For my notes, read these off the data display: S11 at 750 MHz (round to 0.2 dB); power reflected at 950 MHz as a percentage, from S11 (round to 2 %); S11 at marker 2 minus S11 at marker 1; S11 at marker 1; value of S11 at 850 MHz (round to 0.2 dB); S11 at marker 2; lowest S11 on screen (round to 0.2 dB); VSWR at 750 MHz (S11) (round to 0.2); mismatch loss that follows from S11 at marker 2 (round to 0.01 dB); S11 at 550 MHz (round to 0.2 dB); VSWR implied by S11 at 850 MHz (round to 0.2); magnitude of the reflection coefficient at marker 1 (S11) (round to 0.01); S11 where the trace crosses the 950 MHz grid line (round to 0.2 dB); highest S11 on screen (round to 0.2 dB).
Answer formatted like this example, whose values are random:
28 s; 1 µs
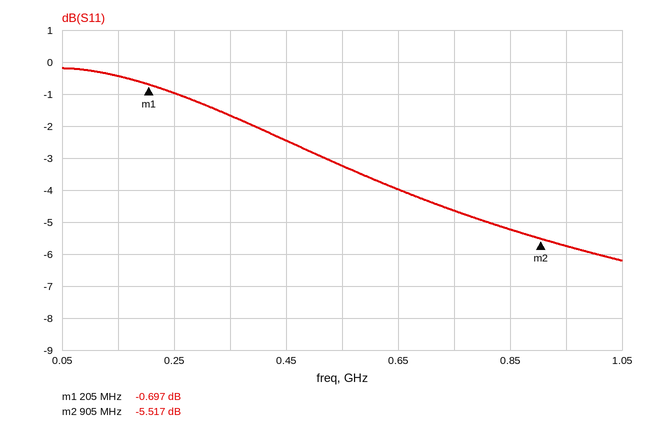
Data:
-4.6 dB; 26 %; -4.820 dB; -0.697 dB; -5.2 dB; -5.517 dB; -6.2 dB; 3.8; 1.43 dB; -3.2 dB; 3.4; 0.92; -5.8 dB; -0.2 dB
